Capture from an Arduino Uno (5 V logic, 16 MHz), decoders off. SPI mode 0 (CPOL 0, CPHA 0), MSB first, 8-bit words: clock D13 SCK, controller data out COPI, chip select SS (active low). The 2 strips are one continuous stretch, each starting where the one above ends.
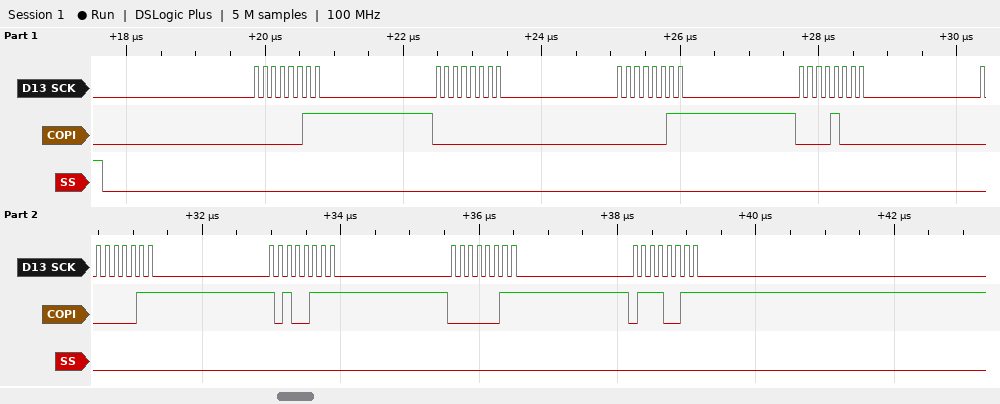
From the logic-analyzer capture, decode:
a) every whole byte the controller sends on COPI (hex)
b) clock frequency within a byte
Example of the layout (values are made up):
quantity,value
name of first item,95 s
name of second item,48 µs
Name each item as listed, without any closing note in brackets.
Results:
quantity,value
every whole byte the controller sends on COPI,0x03 0x00 0x03 0x08 0x03 0xA7 0x03 0x73
clock frequency within a byte,8 MHz
